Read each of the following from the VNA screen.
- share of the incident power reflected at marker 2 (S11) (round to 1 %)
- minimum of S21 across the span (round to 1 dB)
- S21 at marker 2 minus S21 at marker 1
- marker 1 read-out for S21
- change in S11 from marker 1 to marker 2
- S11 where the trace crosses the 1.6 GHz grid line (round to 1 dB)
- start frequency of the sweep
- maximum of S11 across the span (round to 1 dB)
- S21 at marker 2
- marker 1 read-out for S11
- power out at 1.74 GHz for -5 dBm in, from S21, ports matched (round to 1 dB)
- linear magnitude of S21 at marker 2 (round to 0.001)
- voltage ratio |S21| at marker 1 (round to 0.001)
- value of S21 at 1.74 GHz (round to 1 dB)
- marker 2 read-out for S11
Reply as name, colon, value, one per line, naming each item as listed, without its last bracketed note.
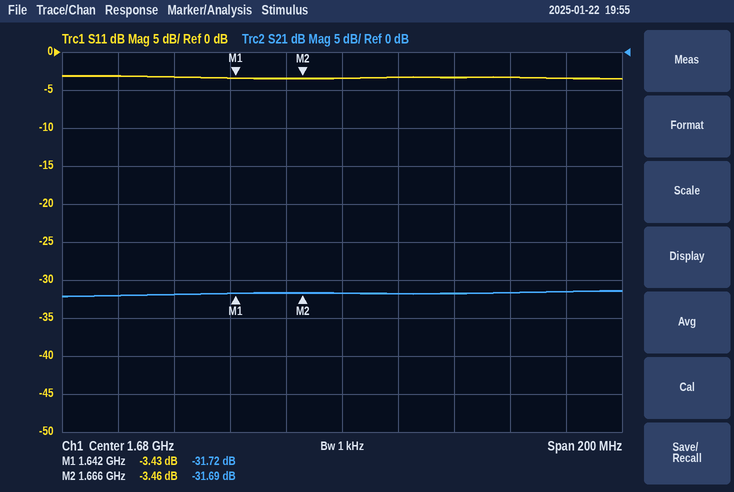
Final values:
share of the incident power reflected at marker 2 (S11): 45 %
minimum of S21 across the span: -32 dB
S21 at marker 2 minus S21 at marker 1: 0.03 dB
marker 1 read-out for S21: -31.72 dB
change in S11 from marker 1 to marker 2: -0.03 dB
S11 where the trace crosses the 1.6 GHz grid line: -3 dB
start frequency of the sweep: 1.58 GHz
maximum of S11 across the span: -3 dB
S21 at marker 2: -31.69 dB
marker 1 read-out for S11: -3.43 dB
power out at 1.74 GHz for -5 dBm in, from S21, ports matched: -37 dBm
linear magnitude of S21 at marker 2: 0.026
voltage ratio |S21| at marker 1: 0.026
value of S21 at 1.74 GHz: -32 dB
marker 2 read-out for S11: -3.46 dB
